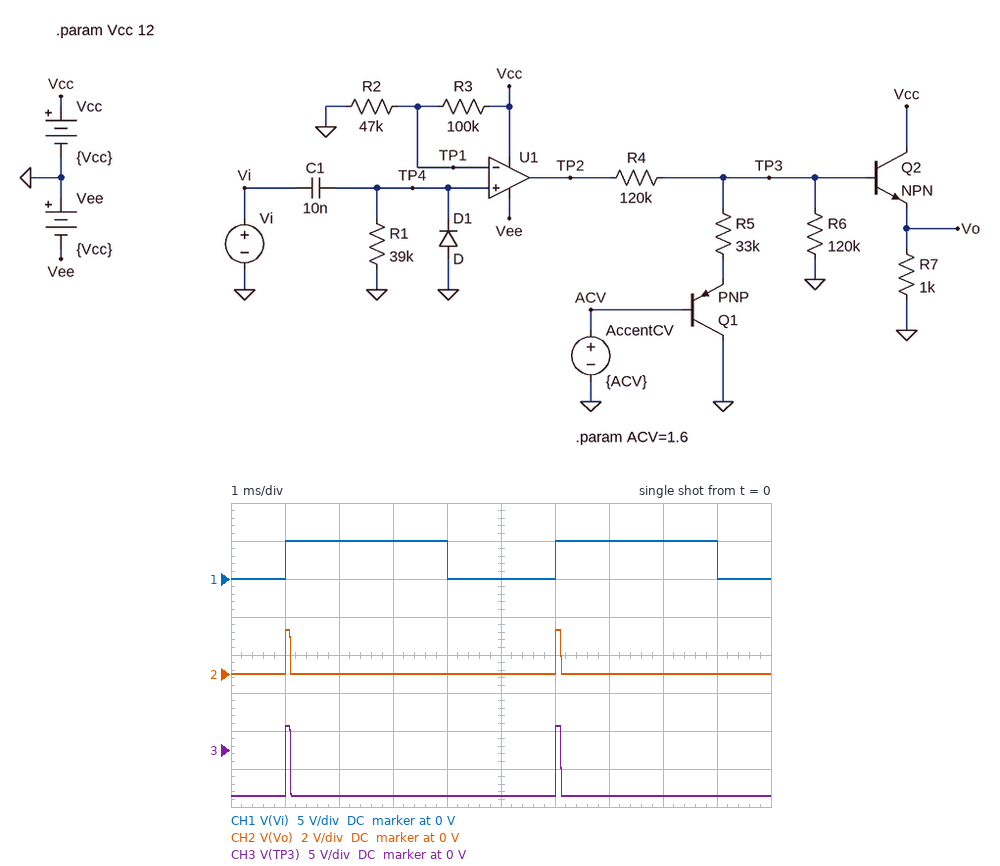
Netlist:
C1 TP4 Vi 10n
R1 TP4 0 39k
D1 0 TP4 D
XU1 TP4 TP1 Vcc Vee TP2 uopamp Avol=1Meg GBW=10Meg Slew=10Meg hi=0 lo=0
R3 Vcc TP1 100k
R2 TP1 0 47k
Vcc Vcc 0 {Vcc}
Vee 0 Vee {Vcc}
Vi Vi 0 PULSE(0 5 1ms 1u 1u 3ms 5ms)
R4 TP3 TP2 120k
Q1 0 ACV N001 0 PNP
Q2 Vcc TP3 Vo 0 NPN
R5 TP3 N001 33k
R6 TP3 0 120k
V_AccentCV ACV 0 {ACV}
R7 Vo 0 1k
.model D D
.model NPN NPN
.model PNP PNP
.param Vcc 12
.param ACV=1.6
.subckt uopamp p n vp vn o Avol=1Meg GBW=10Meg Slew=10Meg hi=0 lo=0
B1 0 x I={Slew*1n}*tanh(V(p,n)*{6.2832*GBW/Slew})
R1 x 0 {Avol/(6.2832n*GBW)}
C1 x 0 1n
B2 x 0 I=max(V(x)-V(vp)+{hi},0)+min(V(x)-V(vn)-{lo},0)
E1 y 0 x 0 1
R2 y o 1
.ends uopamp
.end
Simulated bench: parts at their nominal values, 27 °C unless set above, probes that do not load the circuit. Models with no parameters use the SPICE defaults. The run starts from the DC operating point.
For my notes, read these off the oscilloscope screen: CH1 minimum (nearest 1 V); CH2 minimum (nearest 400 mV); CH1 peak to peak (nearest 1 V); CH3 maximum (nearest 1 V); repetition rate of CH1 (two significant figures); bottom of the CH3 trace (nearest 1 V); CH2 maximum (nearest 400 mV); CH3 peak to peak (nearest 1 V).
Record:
0 V
0 V
5 V
3 V
200 Hz
-6 V
2.4 V
9 V
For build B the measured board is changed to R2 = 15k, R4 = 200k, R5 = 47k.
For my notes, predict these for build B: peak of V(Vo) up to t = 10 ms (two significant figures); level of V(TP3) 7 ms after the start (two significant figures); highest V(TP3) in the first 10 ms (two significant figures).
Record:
1.8 V
-4.5 V
2.6 V
